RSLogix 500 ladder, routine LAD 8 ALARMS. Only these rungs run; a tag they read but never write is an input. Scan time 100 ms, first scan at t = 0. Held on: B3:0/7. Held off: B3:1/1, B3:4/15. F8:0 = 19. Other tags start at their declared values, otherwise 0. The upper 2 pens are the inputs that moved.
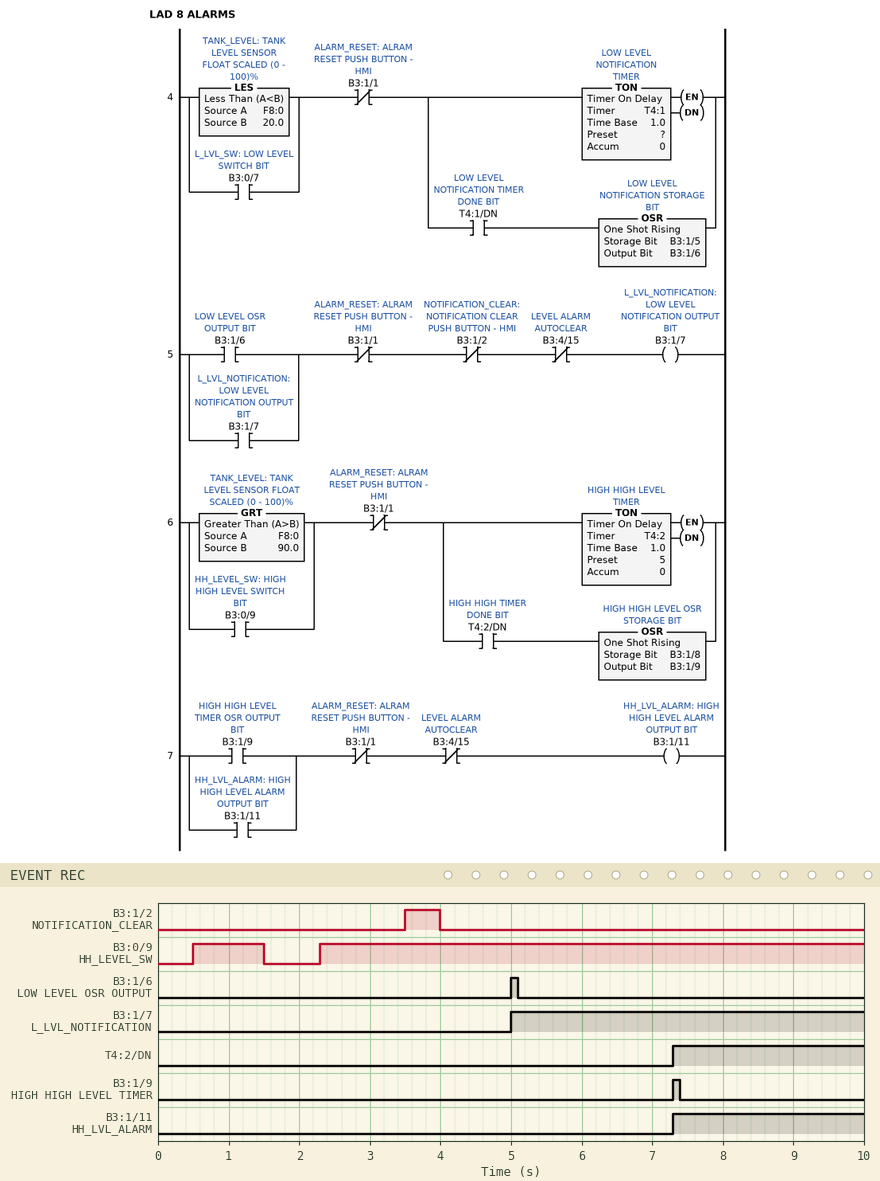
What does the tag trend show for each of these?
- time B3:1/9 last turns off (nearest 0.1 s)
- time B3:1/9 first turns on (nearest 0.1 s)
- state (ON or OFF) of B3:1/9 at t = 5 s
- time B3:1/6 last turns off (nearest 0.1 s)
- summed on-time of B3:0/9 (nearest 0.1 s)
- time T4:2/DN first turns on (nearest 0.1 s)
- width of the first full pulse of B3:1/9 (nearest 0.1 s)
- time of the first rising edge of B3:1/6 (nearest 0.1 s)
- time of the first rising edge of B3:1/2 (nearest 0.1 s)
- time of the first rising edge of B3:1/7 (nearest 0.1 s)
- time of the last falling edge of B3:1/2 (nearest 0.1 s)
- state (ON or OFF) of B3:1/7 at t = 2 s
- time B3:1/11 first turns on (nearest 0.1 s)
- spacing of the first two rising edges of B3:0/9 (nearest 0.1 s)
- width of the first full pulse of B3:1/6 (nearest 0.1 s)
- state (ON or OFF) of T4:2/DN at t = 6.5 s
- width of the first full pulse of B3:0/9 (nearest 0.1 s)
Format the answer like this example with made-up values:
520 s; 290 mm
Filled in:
7.4 s; 7.3 s; OFF; 5.1 s; 8.7 s; 7.3 s; 0.1 s; 5.0 s; 3.5 s; 5.0 s; 4.0 s; OFF; 7.3 s; 1.8 s; 0.1 s; OFF; 1.0 s
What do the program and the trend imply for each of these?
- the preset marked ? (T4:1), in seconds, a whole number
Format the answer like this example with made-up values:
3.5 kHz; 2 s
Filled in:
5 s
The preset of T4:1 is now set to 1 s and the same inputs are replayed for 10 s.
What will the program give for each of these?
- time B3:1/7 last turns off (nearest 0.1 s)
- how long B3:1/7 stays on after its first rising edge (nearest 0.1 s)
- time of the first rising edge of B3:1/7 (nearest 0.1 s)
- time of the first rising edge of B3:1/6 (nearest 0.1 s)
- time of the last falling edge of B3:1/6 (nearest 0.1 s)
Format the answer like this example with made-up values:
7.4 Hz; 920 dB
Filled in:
3.5 s; 2.5 s; 1.0 s; 1.0 s; 1.1 s
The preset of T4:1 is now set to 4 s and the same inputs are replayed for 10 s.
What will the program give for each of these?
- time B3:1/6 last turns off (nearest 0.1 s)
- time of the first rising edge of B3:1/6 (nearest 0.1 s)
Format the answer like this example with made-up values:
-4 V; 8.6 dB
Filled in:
4.1 s; 4.0 s
